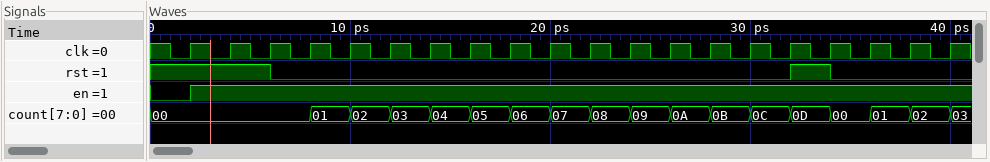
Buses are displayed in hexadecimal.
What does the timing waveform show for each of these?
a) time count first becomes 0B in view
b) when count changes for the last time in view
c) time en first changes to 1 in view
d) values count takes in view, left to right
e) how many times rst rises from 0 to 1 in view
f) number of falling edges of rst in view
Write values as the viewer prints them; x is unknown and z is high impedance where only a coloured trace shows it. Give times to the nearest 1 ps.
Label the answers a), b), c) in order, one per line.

a) 28 ps
b) 40 ps
c) 2 ps
d) 00, 01, 02, 03, 04, 05, 06, 07, 08, 09, 0A, 0B, 0C, 0D, 00, 01, 02, 03
e) 1
f) 2
